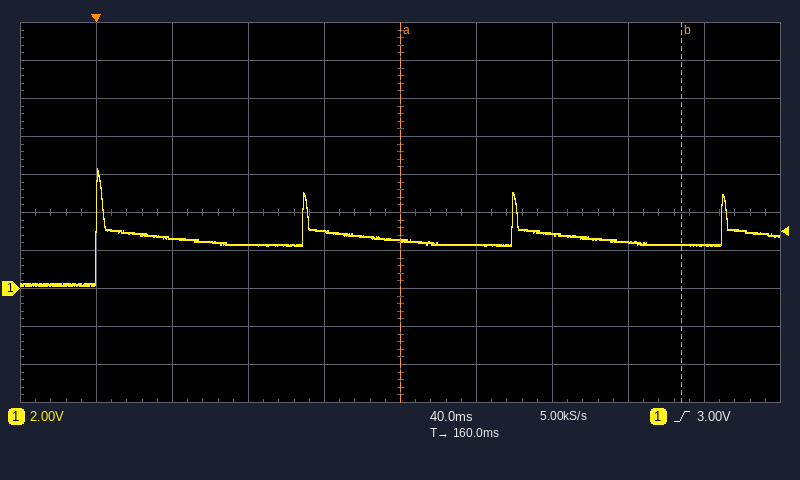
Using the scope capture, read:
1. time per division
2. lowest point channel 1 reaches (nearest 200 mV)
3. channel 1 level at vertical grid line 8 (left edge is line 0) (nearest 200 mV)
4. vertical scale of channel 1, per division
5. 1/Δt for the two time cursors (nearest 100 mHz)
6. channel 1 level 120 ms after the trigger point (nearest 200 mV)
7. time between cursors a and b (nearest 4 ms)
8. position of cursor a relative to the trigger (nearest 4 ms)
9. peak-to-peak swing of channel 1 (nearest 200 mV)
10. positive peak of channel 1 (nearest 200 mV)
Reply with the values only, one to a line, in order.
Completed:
40 ms
200 mV
2.4 V
2 V
6.8 Hz
3.0 V
148 ms
+160 ms
6.2 V
6.4 V
